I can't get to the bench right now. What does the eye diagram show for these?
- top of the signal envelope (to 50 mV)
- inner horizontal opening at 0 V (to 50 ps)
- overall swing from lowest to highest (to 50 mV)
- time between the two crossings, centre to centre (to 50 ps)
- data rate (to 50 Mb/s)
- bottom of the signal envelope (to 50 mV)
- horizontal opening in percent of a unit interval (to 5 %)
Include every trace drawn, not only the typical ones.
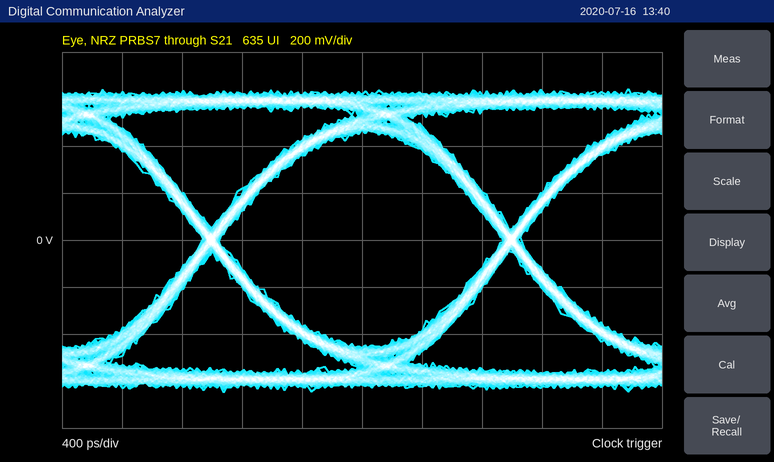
650 mV
1.90 ns
1.30 V
2.00 ns
500 Mb/s
-650 mV
95 %
